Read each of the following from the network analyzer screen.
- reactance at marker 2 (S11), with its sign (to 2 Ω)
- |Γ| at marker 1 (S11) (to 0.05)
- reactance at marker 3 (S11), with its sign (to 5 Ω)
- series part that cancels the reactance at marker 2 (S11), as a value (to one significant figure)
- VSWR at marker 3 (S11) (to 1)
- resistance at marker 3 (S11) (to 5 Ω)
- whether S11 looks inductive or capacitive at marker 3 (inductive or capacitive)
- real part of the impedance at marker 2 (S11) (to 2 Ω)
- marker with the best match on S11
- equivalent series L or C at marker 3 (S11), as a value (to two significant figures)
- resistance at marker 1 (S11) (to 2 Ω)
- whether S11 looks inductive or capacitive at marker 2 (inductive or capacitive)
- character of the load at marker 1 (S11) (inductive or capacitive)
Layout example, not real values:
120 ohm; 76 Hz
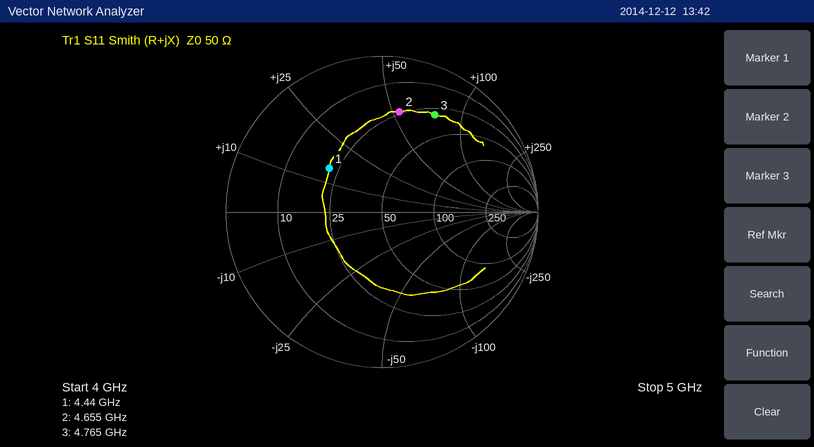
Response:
+54 Ω; 0.45; +75 Ω; 600 fF; 6; 30 Ω; inductive; 24 Ω; marker 1; 2.5 nH; 22 Ω; inductive; inductive
